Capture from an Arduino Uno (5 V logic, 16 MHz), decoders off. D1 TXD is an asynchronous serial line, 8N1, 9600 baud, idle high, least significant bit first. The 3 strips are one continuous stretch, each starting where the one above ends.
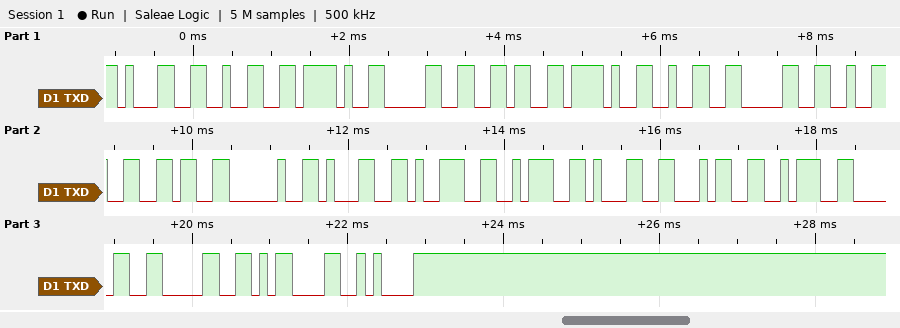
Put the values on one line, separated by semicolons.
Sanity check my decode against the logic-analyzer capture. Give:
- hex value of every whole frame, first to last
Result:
0x31 0x32 0x2F 0x30 0x36 0x2F 0x32 0x30 0x32 0x36 0x20 0x31 0x39 0x3A 0x31 0x34 0x3A 0x30 0x30 0x0D 0x0A
